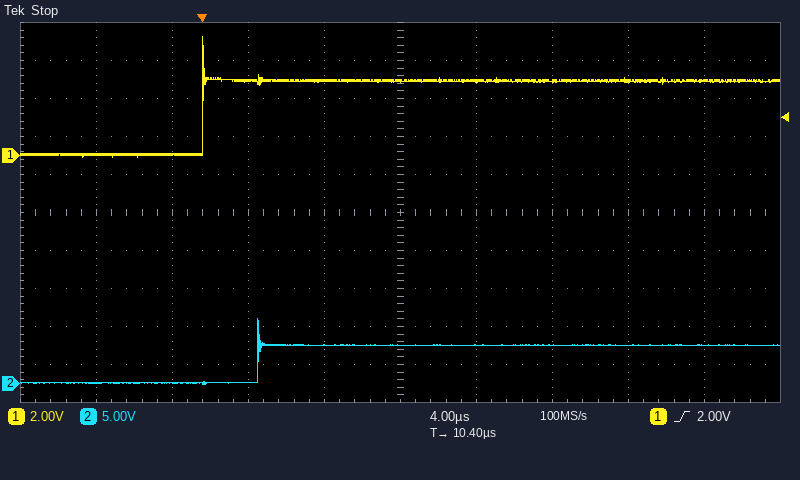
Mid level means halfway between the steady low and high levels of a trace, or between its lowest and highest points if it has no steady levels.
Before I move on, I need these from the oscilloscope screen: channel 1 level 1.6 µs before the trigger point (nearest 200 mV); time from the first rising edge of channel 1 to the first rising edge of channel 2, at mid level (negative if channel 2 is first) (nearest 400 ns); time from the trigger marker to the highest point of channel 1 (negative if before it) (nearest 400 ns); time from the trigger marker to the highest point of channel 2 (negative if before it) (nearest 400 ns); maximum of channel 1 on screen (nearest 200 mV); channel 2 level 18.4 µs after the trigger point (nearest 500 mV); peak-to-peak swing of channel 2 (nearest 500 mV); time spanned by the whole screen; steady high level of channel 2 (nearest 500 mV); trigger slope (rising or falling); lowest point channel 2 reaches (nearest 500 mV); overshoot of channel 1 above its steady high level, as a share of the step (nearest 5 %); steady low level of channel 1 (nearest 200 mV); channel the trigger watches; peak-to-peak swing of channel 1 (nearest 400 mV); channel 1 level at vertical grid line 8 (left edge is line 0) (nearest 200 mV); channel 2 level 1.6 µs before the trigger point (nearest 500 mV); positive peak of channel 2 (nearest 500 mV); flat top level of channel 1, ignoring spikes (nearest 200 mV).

0.0 V
+2.8 µs
0.0 µs
+2.8 µs
6.2 V
5.0 V
8.5 V
40 µs
5.0 V
rising
0.0 V
60 %
0.0 V
channel 1
6.4 V
4.0 V
0.0 V
8.5 V
4.0 V
